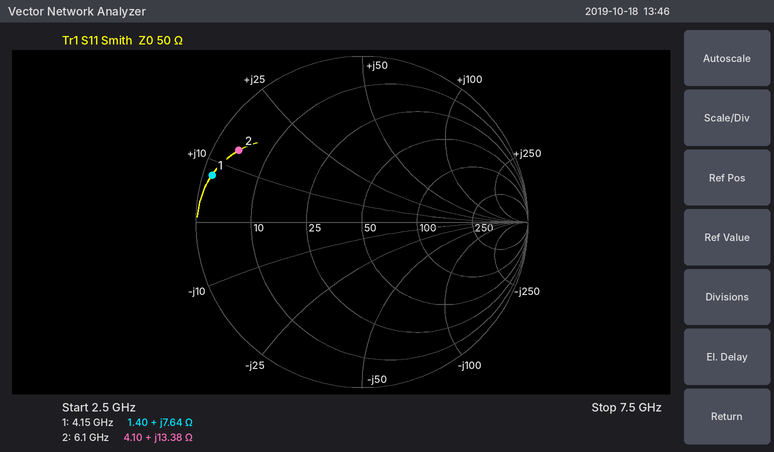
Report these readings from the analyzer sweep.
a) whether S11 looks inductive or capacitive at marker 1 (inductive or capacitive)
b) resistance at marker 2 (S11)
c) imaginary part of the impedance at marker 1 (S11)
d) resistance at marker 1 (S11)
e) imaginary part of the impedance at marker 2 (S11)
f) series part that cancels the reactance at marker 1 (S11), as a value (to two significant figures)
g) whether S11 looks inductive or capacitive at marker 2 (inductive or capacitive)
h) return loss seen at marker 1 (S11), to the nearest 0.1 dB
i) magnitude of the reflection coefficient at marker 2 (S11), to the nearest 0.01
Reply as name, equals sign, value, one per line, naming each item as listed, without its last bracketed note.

whether S11 looks inductive or capacitive at marker 1 = inductive
resistance at marker 2 = 4.10 Ω
imaginary part of the impedance at marker 1 = +7.64 Ω
resistance at marker 1 = 1.40 Ω
imaginary part of the impedance at marker 2 = +13.38 Ω
series part that cancels the reactance at marker 1 (S11), as a value = 5.0 pF
whether S11 looks inductive or capacitive at marker 2 = inductive
return loss seen at marker 1 (S11), to the nearest 0.1 dB = 0.5 dB
magnitude of the reflection coefficient at marker 2 (S11), to the nearest 0.01 = 0.86
